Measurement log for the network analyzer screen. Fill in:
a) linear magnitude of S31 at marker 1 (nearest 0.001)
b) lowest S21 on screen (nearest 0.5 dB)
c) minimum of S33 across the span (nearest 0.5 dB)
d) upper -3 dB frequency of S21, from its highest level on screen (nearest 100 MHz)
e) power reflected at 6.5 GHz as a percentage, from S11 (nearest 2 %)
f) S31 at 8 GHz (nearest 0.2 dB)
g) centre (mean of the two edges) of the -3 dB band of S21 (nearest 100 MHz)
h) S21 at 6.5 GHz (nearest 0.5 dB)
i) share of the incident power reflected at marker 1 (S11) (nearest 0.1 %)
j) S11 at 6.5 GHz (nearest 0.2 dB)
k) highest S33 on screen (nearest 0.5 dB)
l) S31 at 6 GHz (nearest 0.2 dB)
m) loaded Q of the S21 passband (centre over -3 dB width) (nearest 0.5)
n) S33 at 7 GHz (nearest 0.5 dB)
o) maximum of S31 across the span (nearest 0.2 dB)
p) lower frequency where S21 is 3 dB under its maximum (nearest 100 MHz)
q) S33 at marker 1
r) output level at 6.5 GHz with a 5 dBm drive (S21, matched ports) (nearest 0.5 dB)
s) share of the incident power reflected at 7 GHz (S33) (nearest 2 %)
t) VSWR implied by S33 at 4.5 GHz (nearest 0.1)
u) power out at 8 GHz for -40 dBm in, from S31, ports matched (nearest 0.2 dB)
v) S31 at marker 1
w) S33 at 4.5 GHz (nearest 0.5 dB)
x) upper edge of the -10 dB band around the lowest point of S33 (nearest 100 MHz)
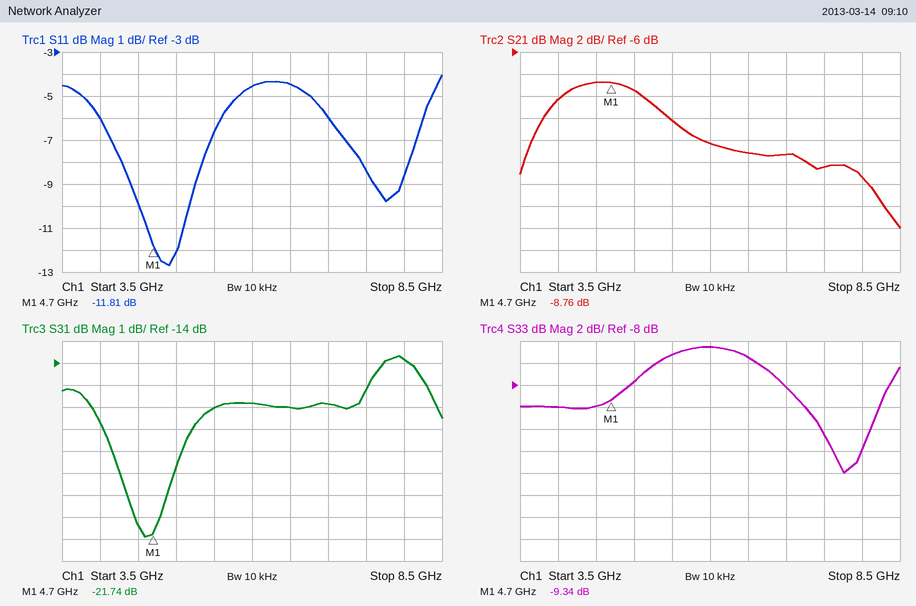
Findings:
0.082
-22.0 dB
-16.0 dB
5.4 GHz
36 %
-13.8 dB
4.6 GHz
-15.0 dB
6.6 %
-4.4 dB
-4.5 dB
-15.8 dB
3.0
-8.0 dB
-13.6 dB
3.8 GHz
-9.34 dB
-10.0 dBm
16 %
1.9
-53.8 dBm
-21.74 dB
-10.0 dB
8.2 GHz
